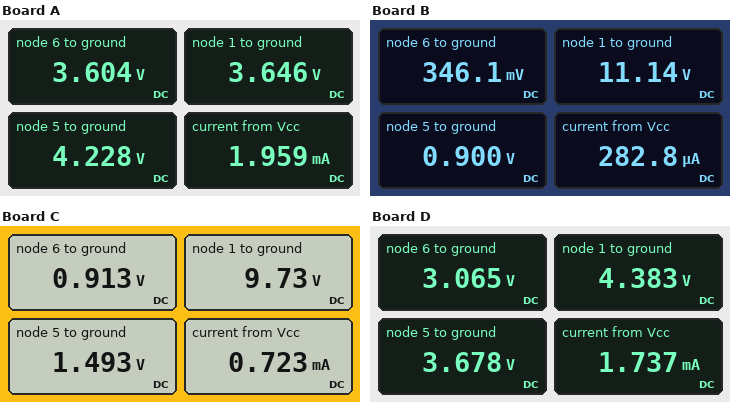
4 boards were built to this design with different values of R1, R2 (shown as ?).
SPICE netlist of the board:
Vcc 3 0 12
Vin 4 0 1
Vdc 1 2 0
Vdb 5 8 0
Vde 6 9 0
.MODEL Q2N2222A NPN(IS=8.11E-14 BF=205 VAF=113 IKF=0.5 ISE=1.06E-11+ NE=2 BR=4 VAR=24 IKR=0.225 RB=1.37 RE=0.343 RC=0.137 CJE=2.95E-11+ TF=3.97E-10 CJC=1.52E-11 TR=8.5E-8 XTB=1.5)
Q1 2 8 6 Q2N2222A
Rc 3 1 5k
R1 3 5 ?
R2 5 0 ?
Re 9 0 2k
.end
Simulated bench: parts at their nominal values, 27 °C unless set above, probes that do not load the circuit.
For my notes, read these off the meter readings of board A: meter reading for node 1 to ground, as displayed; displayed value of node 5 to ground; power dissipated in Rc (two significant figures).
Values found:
3.646 V
4.228 V
14 mW
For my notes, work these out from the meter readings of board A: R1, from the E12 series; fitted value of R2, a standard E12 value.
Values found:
27 kΩ
27 kΩ
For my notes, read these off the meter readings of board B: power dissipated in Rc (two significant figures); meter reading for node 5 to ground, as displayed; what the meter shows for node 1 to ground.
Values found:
150 µW
0.900 V
11.14 V
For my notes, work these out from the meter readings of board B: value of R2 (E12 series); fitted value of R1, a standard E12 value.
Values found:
8.2 kΩ
100 kΩ
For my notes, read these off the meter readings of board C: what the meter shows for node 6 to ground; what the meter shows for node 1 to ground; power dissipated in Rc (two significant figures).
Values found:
0.913 V
9.73 V
1.0 mW
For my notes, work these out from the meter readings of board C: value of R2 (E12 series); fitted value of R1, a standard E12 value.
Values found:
5.6 kΩ
39 kΩ
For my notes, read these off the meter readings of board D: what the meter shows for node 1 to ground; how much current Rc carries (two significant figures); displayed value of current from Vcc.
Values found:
4.383 V
1.5 mA
1.737 mA
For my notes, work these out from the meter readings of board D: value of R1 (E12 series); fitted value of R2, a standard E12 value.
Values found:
39 kΩ
18 kΩ
